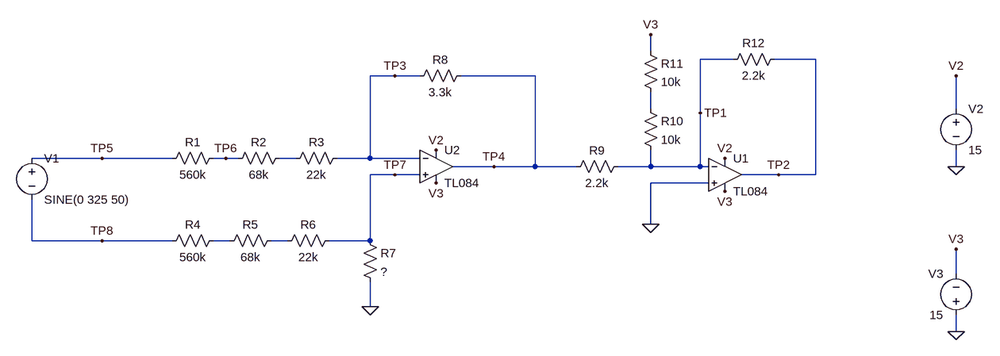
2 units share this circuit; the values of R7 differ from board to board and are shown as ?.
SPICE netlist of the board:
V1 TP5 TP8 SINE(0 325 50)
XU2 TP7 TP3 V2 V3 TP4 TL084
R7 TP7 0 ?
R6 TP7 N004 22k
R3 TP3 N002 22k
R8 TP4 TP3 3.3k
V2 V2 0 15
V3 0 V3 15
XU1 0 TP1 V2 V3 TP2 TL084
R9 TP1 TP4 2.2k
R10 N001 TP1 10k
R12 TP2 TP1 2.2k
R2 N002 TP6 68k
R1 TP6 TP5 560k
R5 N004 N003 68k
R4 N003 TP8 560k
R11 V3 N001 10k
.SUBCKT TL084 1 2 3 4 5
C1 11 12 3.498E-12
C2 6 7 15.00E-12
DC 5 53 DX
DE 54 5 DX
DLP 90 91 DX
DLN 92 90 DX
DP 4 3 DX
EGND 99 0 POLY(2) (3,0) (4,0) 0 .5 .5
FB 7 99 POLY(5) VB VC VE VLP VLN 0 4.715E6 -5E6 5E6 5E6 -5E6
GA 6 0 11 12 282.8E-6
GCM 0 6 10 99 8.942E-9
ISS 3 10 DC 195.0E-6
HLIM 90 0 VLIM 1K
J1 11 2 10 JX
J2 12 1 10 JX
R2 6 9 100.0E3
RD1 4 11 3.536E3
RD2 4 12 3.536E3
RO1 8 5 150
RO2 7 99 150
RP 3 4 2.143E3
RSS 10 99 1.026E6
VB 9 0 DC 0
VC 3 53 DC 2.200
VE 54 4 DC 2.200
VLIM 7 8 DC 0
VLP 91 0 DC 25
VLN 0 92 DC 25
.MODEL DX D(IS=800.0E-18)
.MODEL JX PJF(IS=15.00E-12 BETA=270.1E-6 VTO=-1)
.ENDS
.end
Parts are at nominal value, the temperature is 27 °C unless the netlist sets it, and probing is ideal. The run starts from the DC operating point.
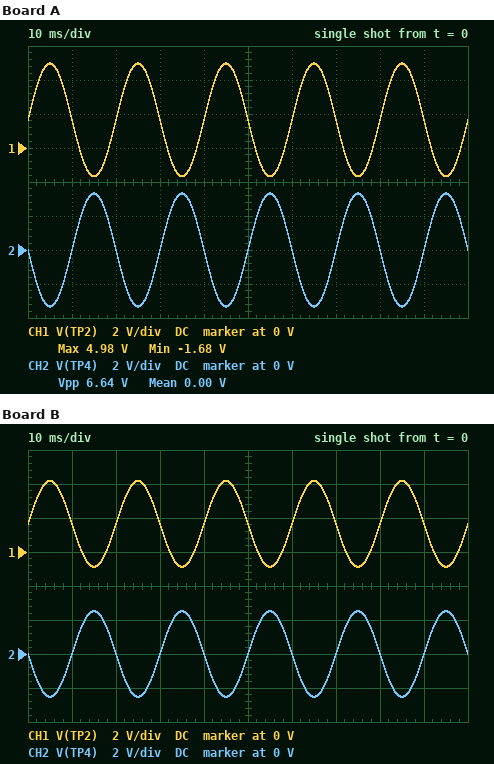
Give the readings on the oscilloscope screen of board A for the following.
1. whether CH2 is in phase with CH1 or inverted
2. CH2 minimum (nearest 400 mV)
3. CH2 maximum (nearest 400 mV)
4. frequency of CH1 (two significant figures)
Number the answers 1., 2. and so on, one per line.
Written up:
1. inverted
2. -3.2 V
3. 3.2 V
4. 50 Hz
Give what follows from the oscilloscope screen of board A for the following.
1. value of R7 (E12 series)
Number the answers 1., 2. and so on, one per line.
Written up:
1. 10 kΩ
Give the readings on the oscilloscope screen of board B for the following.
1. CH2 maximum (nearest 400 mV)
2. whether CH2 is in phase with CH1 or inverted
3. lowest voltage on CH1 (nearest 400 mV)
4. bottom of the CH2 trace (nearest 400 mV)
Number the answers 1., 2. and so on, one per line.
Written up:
1. 2.4 V
2. inverted
3. -800 mV
4. -2.4 V
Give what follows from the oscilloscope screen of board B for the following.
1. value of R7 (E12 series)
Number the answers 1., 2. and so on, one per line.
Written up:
1. 6.8 kΩ
